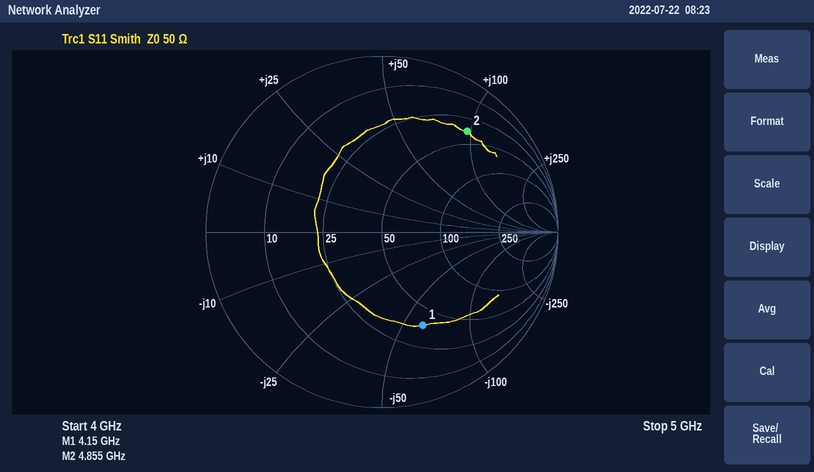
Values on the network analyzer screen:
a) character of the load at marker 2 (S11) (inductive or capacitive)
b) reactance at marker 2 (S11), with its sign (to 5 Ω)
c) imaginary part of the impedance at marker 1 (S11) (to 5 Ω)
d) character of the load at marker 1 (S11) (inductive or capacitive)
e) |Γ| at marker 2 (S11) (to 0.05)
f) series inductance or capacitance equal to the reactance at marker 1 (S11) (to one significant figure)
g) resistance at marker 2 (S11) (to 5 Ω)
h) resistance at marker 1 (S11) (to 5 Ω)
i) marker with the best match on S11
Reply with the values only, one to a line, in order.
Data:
inductive
+95 Ω
-60 Ω
capacitive
0.75
600 fF
35 Ω
40 Ω
marker 1
